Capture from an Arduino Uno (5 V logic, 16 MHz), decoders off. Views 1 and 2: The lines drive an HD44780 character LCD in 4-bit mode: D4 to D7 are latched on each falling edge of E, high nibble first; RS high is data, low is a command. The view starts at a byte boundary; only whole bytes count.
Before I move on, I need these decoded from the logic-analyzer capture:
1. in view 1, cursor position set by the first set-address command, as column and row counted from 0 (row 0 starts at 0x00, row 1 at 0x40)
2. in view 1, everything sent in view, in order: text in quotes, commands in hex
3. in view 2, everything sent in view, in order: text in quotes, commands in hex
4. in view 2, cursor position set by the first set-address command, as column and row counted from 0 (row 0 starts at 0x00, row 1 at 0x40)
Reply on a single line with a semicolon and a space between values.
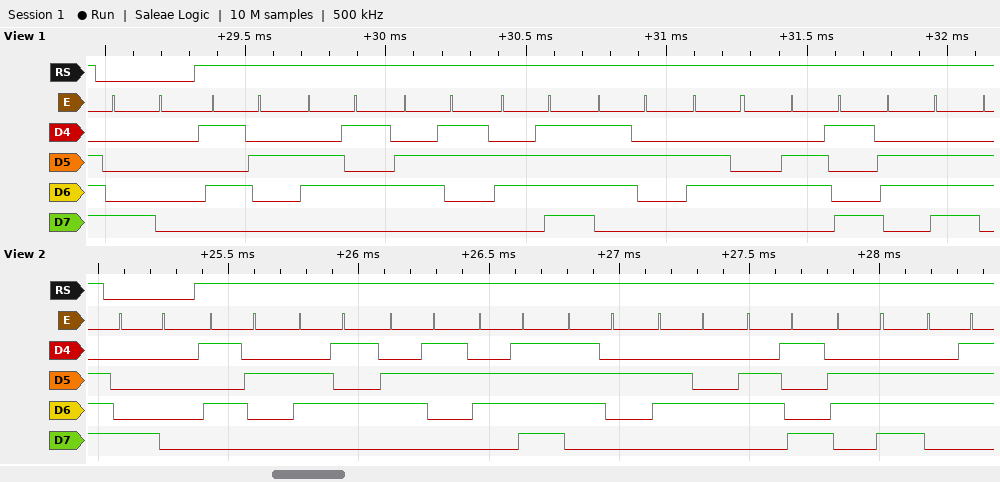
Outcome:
column 0, row 0; 0x80 "Recordin"; 0x80 "Recording"; column 0, row 0
